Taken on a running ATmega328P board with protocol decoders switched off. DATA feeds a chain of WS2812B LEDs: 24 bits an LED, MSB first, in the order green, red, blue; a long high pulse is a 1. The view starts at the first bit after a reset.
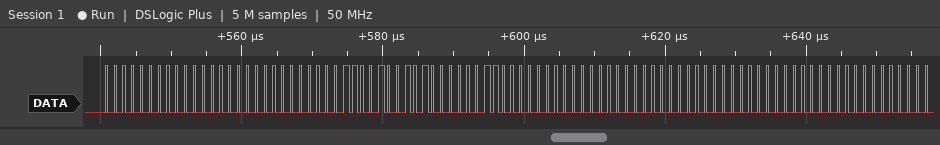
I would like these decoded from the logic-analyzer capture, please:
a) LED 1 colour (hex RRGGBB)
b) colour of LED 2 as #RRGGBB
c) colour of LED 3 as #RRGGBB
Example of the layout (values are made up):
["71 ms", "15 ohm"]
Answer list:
["#000000", "#281918", "#000000"]
